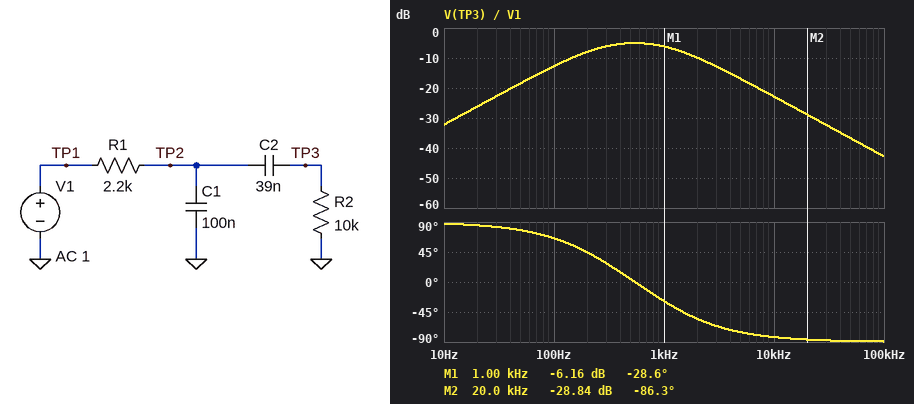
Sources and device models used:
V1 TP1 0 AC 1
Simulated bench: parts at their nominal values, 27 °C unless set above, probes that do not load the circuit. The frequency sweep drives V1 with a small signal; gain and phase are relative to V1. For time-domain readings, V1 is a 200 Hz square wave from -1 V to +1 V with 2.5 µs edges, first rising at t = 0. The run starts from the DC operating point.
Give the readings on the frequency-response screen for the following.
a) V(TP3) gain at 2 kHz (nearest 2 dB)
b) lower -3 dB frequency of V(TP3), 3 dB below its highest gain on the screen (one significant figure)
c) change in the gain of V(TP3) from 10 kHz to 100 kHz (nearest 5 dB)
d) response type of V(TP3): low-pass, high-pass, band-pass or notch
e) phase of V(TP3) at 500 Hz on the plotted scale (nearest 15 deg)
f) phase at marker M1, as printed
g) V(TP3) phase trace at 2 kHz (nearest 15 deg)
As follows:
-10 dB
200 Hz
-20 dB
band-pass
0 deg
-28.6 deg
-60 deg
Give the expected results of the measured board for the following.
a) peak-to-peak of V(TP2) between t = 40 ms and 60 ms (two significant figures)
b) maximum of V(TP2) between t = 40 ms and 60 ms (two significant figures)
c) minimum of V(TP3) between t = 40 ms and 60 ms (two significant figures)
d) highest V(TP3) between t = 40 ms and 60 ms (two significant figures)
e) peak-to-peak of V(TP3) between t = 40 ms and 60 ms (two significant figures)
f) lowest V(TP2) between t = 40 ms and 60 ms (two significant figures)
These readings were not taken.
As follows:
2.0 V
990 mV
-860 mV
860 mV
1.7 V
-990 mV
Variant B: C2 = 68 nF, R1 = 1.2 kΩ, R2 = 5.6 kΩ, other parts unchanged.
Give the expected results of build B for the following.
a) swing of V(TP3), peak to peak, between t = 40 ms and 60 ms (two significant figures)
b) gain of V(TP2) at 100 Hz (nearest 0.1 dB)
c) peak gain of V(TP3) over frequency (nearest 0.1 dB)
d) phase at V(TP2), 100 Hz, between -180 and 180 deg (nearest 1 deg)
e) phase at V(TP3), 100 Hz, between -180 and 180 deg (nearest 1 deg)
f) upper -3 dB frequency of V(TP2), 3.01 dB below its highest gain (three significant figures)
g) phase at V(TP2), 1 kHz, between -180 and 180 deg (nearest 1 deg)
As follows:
2.1 V
-0.2 dB
-3.7 dB
-7 deg
70 deg
931 Hz
-35 deg
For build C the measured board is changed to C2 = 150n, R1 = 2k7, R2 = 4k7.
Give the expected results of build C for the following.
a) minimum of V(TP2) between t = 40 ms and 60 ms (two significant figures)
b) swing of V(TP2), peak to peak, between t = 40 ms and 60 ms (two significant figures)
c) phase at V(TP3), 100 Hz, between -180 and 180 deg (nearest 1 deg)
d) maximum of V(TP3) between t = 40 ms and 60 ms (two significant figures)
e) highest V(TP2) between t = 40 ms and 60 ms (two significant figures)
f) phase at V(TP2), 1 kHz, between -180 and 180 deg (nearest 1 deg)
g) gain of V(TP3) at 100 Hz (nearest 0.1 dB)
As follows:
-890 mV
1.8 V
47 deg
740 mV
890 mV
-50 deg
-9.1 dB
